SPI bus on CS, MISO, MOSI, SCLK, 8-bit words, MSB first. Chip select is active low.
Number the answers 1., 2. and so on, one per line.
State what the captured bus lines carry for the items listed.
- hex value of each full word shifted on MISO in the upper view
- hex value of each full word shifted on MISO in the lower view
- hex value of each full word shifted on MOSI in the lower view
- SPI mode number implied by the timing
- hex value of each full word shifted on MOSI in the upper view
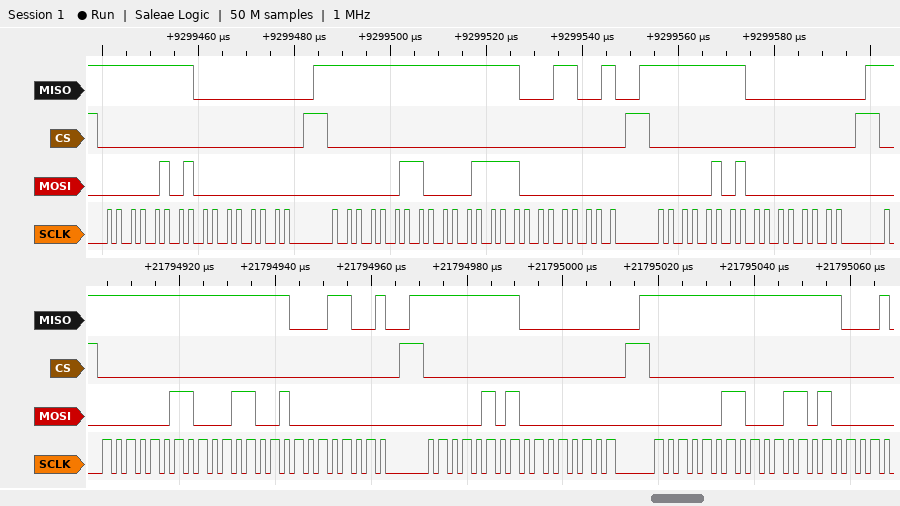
1. FF, 00, FF, FF, 19, FF, 00
2. FF, FF, 19, FF, 00, FF, FF
3. 03, 19, 00, 05, 00, 03, 1A
4. 0
5. 05, 00, 03, 0F, 00, 05, 00
